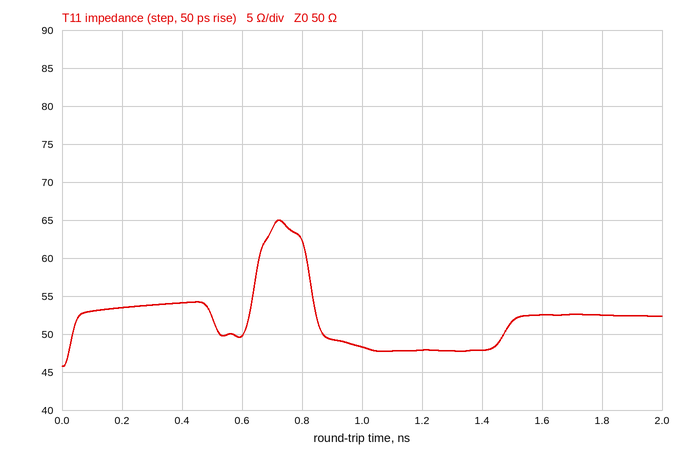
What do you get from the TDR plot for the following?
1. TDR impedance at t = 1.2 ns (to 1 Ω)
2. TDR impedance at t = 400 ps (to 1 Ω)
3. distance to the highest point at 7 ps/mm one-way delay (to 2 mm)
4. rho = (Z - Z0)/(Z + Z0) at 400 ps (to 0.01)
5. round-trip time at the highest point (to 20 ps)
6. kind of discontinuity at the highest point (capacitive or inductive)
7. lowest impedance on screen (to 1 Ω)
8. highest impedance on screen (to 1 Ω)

48 Ω
54 Ω
52 mm
+0.04
720 ps
inductive
46 Ω
65 Ω
